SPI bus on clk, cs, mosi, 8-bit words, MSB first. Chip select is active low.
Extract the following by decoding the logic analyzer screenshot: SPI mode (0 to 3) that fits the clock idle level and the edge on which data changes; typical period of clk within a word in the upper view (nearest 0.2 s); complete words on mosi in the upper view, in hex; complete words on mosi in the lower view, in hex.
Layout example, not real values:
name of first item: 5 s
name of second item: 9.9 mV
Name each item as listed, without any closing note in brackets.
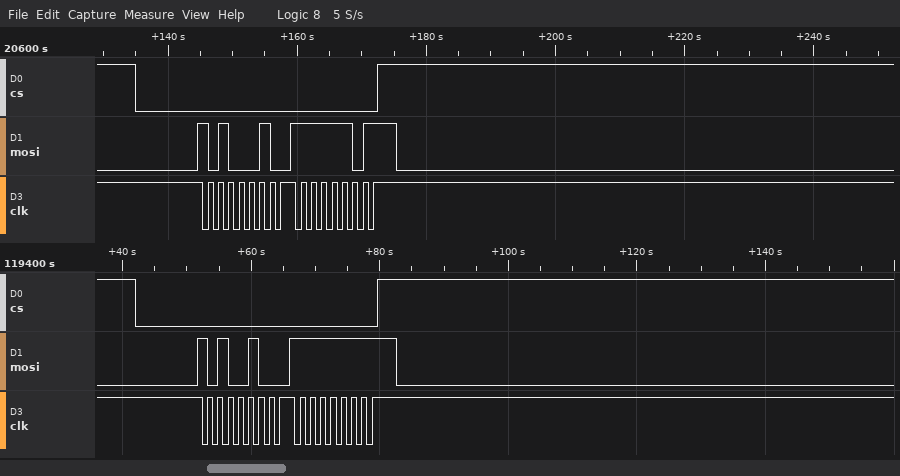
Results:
SPI mode (0 to 3) that fits the clock idle level and the edge on which data changes: 2
typical period of clk within a word in the upper view: 1.6 s
complete words on mosi in the upper view, in hex: A2, FD
complete words on mosi in the lower view, in hex: A4, FF
